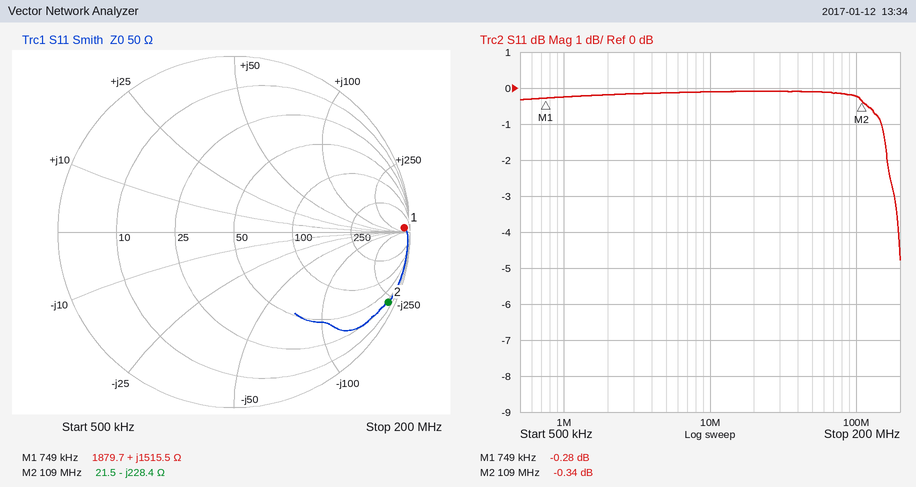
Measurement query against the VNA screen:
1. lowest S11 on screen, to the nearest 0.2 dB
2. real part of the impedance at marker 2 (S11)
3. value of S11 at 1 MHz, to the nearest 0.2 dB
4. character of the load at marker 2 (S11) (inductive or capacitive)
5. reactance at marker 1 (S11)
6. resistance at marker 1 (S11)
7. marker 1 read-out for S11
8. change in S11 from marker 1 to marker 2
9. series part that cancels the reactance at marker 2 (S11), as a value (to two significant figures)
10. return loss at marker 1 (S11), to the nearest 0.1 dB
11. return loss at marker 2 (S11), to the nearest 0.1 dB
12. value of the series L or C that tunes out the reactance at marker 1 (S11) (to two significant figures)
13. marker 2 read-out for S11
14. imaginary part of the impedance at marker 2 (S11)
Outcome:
-4.8 dB
21.5 Ω
-0.2 dB
capacitive
+1515.5 Ω
1879.7 Ω
-0.28 dB
-0.06 dB
330 nH
0.3 dB
0.3 dB
140 pF
-0.34 dB
-228.4 Ω
